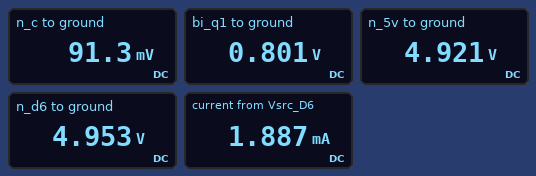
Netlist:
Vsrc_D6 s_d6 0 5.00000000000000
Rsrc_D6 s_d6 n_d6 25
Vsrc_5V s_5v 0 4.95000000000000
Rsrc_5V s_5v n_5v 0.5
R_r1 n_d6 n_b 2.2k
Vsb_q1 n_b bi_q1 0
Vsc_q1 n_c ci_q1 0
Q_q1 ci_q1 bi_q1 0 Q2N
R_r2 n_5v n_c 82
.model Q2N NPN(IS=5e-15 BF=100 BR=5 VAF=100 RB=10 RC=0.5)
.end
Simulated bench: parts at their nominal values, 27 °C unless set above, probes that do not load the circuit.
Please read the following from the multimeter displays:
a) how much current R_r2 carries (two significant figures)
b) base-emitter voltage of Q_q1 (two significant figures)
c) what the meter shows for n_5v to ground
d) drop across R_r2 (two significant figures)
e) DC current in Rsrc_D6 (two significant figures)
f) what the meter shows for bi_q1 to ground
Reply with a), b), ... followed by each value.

a) 59 mA
b) 800 mV
c) 4.921 V
d) 4.8 V
e) 1.9 mA
f) 0.801 V
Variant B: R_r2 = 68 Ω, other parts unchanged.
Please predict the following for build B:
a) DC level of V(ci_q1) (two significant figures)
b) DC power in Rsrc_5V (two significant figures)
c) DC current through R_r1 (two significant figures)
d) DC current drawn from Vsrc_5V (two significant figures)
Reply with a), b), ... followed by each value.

a) 100 mV
b) 2.5 mW
c) 1.9 mA
d) 71 mA
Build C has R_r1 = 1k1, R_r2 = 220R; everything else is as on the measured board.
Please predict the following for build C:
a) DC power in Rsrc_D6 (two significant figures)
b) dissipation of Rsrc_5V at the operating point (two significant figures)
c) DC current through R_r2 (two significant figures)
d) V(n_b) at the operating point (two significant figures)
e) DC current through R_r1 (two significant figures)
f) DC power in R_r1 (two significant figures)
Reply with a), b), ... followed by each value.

a) 350 µW
b) 250 µW
c) 22 mA
d) 810 mV
e) 3.7 mA
f) 15 mW
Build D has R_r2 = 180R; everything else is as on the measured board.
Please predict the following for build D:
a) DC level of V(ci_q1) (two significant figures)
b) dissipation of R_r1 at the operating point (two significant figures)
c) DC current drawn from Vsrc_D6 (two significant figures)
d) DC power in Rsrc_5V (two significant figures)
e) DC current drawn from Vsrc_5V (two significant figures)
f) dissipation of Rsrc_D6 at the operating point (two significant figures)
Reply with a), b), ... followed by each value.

a) 54 mV
b) 7.9 mW
c) 1.9 mA
d) 370 µW
e) 27 mA
f) 90 µW
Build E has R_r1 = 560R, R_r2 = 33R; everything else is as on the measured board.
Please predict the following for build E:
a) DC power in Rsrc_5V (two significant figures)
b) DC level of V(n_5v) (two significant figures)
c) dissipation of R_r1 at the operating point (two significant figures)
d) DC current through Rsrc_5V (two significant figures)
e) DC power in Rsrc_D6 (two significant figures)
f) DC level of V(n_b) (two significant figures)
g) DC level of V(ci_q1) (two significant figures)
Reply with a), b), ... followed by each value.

a) 10 mW
b) 4.9 V
c) 28 mW
d) 140 mA
e) 1.2 mW
f) 880 mV
g) 120 mV
